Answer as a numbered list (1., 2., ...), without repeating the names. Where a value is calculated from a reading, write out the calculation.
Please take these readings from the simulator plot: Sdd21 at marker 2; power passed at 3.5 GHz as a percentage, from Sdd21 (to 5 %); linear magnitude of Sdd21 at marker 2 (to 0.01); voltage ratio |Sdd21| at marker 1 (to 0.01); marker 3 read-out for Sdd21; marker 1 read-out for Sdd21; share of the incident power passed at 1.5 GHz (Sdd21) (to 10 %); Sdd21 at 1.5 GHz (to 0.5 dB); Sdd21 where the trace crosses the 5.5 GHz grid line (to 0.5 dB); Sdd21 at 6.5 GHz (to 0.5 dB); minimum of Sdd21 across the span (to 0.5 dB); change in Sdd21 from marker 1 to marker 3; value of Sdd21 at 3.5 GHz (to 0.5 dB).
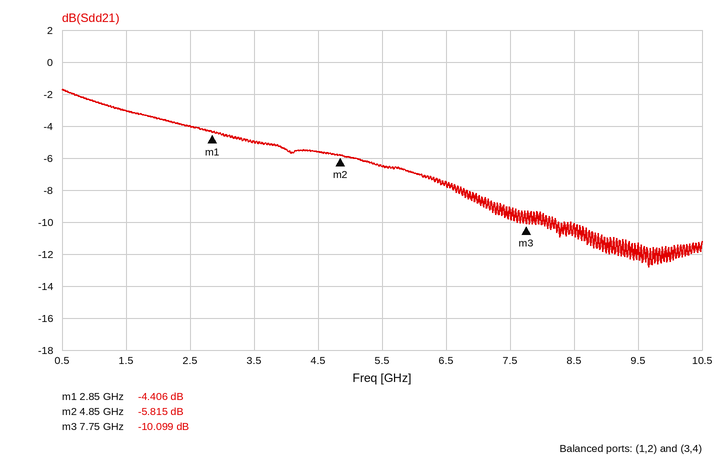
1. -5.815 dB
2. 10^(-5/10) ≈ 31.6 %, so 30 % to the nearest 5 %
3. 10^(-5.815/20) ≈ 0.51
4. 10^(-4.406/20) ≈ 0.60
5. -10.099 dB
6. -4.406 dB
7. 10^(-3/10) ≈ 50 %
8. -3.0 dB
9. -6.5 dB
10. -7.5 dB
11. -13.0 dB
12. -10.099 − (-4.406) = -5.693 dB
13. -5.0 dB
